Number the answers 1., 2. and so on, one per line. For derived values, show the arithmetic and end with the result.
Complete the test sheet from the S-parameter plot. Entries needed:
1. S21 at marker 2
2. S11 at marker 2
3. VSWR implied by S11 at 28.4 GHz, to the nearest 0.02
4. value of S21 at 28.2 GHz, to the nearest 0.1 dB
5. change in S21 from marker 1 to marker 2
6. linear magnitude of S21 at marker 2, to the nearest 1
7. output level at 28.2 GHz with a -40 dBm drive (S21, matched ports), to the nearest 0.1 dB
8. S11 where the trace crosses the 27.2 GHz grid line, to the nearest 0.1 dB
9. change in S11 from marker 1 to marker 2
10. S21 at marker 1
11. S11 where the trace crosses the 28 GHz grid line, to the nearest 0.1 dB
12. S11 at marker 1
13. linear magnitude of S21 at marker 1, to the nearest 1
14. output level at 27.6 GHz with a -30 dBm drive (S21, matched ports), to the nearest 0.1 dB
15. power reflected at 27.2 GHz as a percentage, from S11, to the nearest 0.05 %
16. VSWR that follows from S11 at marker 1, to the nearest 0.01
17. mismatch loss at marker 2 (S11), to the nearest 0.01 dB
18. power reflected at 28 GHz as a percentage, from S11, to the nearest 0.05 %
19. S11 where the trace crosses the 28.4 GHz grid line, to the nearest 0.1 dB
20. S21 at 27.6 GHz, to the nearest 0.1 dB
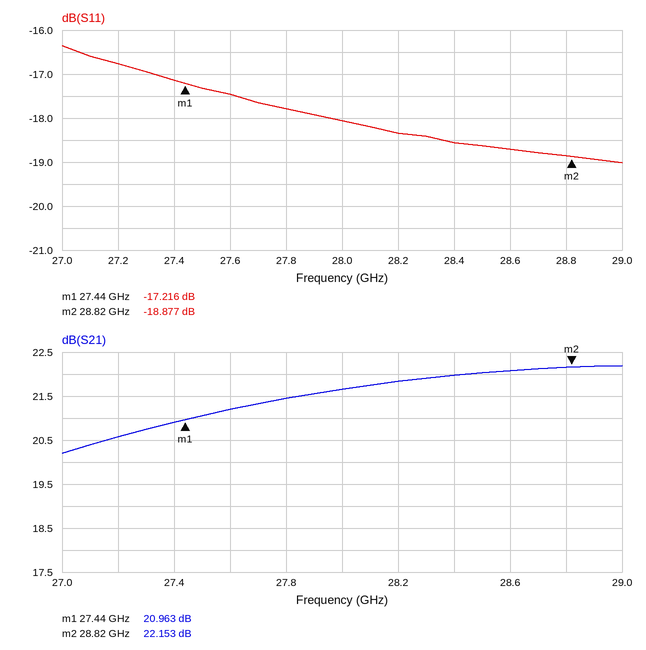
1. 22.153 dB
2. -18.877 dB
3. |Γ| = 10^(-18.6/20) = 0.1175; VSWR = (1 + 0.1175)/(1 − 0.1175) ≈ 1.27, so 1.26 to the nearest 0.02
4. 21.8 dB
5. 22.153 − (20.963) = 1.190 dB
6. 10^(22.153/20) ≈ 13
7. -40 dBm + (21.8 dB) = -18.2 dBm
8. -16.8 dB
9. -18.877 − (-17.216) = -1.661 dB
10. 20.963 dB
11. -18.1 dB
12. -17.216 dB
13. 10^(20.963/20) ≈ 11
14. -30 dBm + (21.2 dB) = -8.8 dBm
15. 10^(-16.8/10) ≈ 2.09 %, so 2.10 % to the nearest 0.05 %
16. (1 + 0.1378)/(1 − 0.1378) ≈ 1.32
17. −10 log10(1 − 10^(-18.877/10)) ≈ 0.06 dB
18. 10^(-18.1/10) ≈ 1.55 %
19. -18.6 dB
20. 21.2 dB
